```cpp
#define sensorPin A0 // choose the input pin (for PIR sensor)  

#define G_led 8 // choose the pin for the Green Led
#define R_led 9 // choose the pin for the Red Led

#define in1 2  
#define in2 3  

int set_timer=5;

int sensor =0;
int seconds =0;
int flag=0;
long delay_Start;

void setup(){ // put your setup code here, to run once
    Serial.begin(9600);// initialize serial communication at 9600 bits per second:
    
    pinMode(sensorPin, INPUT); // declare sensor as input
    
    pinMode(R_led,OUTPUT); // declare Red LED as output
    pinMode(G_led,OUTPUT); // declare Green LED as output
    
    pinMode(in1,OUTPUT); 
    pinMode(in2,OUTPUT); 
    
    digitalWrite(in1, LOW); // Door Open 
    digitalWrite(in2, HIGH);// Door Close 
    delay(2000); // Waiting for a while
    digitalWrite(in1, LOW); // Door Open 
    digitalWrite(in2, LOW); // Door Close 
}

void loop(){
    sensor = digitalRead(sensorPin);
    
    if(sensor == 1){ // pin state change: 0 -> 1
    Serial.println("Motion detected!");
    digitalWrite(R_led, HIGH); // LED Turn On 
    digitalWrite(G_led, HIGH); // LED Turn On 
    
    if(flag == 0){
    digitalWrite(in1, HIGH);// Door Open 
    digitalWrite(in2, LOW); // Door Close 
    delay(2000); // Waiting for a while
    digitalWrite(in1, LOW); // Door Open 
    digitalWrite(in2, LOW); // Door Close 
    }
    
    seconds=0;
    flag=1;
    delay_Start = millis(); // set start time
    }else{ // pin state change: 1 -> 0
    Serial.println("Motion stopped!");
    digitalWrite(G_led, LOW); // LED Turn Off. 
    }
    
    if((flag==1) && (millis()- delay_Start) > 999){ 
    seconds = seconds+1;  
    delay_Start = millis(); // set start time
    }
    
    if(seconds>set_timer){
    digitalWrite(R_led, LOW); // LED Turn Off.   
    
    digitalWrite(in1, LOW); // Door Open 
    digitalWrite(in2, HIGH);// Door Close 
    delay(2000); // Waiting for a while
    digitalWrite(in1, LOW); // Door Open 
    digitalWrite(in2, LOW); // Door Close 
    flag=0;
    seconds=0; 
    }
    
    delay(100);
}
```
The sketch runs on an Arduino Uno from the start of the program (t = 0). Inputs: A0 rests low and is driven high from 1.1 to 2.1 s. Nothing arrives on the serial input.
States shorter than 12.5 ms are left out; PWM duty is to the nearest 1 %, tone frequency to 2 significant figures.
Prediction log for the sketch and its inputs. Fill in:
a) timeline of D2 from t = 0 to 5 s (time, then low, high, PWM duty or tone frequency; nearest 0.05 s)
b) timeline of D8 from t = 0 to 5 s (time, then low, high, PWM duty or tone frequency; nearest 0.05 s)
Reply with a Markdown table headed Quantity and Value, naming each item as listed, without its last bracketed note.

| Quantity | Value |
|---|---|
| timeline of D2 from t = 0 to 5 s | 0 s low; 2 s high; 4 s low |
| timeline of D8 from t = 0 to 5 s | 0 s low; 2 s high; 4.1 s low |
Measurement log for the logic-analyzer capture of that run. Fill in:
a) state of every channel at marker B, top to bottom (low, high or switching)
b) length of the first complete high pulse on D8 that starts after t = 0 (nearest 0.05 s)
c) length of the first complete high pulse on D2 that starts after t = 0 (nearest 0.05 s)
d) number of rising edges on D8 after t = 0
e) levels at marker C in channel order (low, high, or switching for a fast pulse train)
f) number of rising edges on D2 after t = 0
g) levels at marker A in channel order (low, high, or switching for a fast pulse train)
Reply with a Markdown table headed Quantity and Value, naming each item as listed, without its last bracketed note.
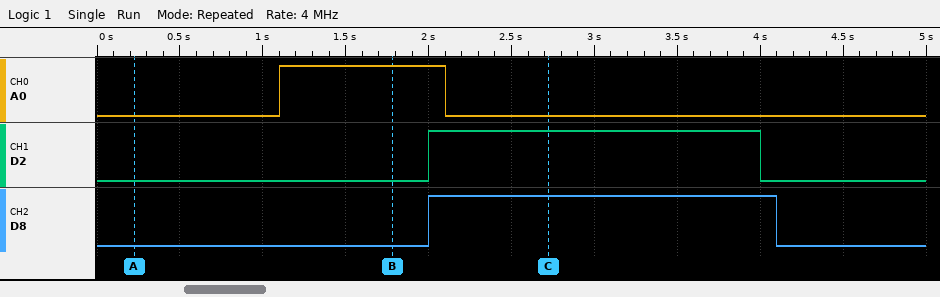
| Quantity | Value |
|---|---|
| state of every channel at marker B, top to bottom | A0 high, D2 low, D8 low |
| length of the first complete high pulse on D8 that starts after t = 0 | 2.10 s |
| length of the first complete high pulse on D2 that starts after t = 0 | 2.00 s |
| number of rising edges on D8 after t = 0 | 1 |
| levels at marker C in channel order | A0 low, D2 high, D8 high |
| number of rising edges on D2 after t = 0 | 1 |
| levels at marker A in channel order | A0 low, D2 low, D8 low |
